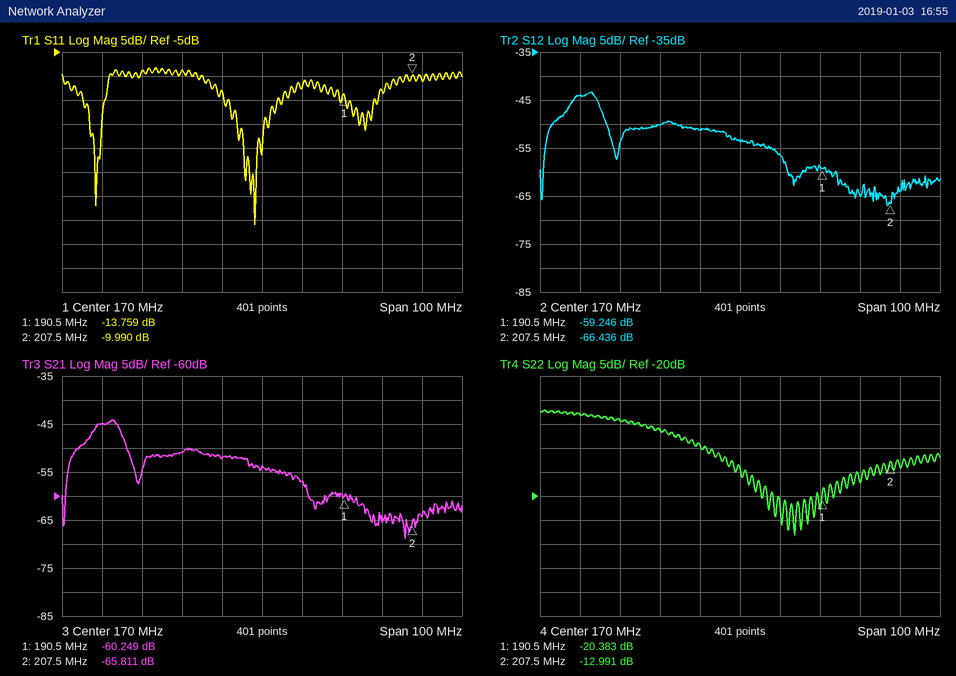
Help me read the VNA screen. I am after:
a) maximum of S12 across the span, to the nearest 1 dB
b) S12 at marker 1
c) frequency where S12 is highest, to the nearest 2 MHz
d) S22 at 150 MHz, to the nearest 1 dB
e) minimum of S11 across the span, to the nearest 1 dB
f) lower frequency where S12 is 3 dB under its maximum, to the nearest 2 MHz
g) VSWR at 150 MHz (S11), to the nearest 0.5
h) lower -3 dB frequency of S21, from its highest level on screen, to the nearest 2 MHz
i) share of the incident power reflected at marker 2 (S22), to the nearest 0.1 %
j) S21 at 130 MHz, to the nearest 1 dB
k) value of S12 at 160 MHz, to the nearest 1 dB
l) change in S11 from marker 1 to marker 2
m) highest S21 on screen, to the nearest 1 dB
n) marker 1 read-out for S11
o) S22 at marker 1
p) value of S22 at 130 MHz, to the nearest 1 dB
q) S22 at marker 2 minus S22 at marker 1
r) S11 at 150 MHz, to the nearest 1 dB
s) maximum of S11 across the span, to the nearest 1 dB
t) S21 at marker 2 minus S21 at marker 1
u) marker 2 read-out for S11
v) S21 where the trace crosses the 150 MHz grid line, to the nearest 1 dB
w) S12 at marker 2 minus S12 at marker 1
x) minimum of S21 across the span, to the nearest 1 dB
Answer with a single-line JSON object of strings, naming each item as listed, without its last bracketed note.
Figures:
{"maximum of S12 across the span, to the nearest 1 dB": "-43 dB", "S12 at marker 1": "-59.246 dB", "frequency where S12 is highest, to the nearest 2 MHz": "132 MHz", "S22 at 150 MHz, to the nearest 1 dB": "-6 dB", "minimum of S11 across the span, to the nearest 1 dB": "-41 dB", "lower frequency where S12 is 3 dB under its maximum, to the nearest 2 MHz": "128 MHz", "VSWR at 150 MHz (S11), to the nearest 0.5": "2.0", "lower -3 dB frequency of S21, from its highest level on screen, to the nearest 2 MHz": "128 MHz", "share of the incident power reflected at marker 2 (S22), to the nearest 0.1 %": "5.0 %", "S21 at 130 MHz, to the nearest 1 dB": "-45 dB", "value of S12 at 160 MHz, to the nearest 1 dB": "-51 dB", "change in S11 from marker 1 to marker 2": "3.769 dB", "highest S21 on screen, to the nearest 1 dB": "-44 dB", "marker 1 read-out for S11": "-13.759 dB", "S22 at marker 1": "-20.383 dB", "value of S22 at 130 MHz, to the nearest 1 dB": "-3 dB", "S22 at marker 2 minus S22 at marker 1": "7.392 dB", "S11 at 150 MHz, to the nearest 1 dB": "-9 dB", "maximum of S11 across the span, to the nearest 1 dB": "-8 dB", "S21 at marker 2 minus S21 at marker 1": "-5.562 dB", "marker 2 read-out for S11": "-9.990 dB", "S21 where the trace crosses the 150 MHz grid line, to the nearest 1 dB": "-51 dB", "S12 at marker 2 minus S12 at marker 1": "-7.190 dB", "minimum of S21 across the span, to the nearest 1 dB": "-69 dB"}
